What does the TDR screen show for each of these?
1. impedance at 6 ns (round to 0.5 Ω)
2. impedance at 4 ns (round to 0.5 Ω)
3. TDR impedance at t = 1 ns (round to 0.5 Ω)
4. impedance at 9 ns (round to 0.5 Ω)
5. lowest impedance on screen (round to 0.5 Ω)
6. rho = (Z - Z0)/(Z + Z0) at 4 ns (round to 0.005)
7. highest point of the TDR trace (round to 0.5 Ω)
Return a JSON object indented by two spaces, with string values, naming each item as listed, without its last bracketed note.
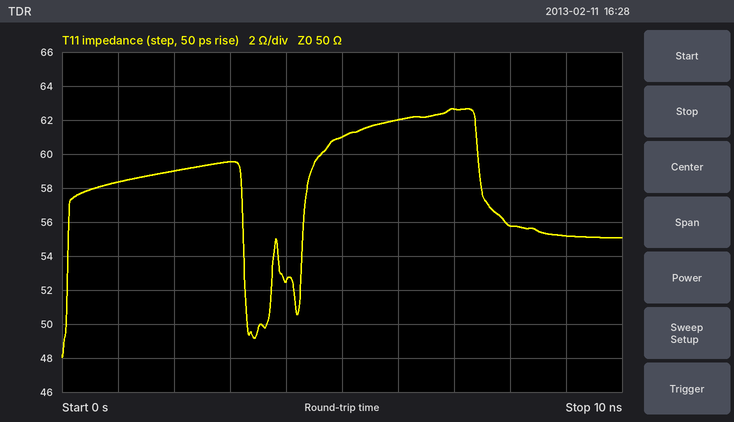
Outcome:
{
  "impedance at 6 ns": "62.0 Ω",
  "impedance at 4 ns": "52.5 Ω",
  "TDR impedance at t = 1 ns": "58.5 Ω",
  "impedance at 9 ns": "55.0 Ω",
  "lowest impedance on screen": "48.0 Ω",
  "rho = (Z - Z0)/(Z + Z0) at 4 ns": "+0.025",
  "highest point of the TDR trace": "62.5 Ω"
}
